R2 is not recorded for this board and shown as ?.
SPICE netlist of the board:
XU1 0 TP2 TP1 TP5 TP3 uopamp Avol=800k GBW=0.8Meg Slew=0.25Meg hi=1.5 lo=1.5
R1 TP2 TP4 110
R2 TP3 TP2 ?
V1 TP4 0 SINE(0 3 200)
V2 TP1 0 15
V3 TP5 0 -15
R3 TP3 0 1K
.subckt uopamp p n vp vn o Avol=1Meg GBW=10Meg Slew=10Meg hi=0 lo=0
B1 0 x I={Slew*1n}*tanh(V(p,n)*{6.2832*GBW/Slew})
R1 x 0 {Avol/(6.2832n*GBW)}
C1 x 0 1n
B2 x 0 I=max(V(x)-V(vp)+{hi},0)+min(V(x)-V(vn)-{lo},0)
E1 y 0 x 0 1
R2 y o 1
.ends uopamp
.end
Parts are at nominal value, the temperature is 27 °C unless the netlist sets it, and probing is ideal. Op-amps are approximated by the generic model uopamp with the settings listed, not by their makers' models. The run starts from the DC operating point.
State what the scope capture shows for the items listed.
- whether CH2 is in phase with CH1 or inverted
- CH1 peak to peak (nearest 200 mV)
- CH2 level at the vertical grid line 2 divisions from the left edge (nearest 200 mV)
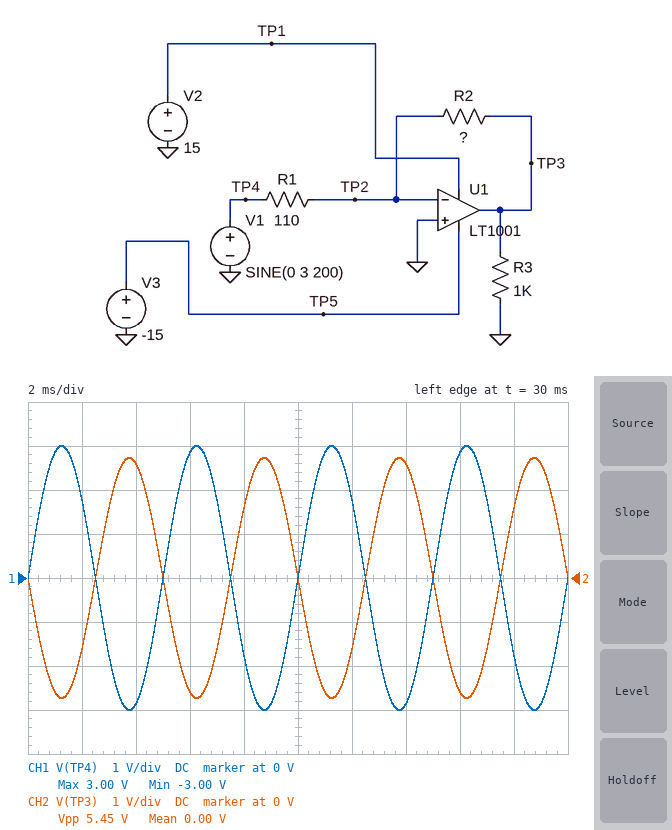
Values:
inverted
6.0 V
2.6 V
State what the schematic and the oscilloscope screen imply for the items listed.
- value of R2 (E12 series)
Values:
100 Ω
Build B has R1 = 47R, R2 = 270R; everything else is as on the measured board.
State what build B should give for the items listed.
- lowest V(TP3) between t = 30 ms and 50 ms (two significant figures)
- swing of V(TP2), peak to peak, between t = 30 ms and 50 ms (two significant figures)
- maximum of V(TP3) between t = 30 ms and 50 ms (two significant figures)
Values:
-13 V
1.1 V
13 V
